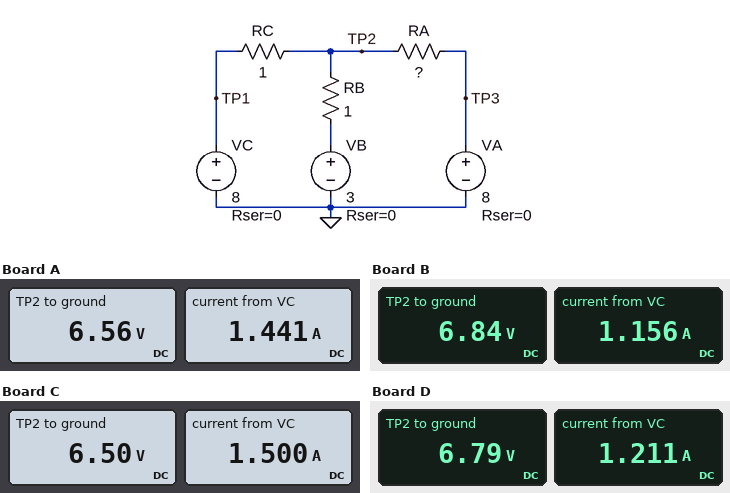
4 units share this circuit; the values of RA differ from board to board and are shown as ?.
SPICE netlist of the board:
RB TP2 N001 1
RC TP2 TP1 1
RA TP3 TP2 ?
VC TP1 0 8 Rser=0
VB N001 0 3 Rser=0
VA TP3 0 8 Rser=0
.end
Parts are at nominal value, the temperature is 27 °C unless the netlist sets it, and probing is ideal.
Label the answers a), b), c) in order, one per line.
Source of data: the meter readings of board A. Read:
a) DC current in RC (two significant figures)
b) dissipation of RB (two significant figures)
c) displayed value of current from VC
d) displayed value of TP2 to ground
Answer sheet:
a) 1.4 A
b) 13 W
c) 1.441 A
d) 6.56 V
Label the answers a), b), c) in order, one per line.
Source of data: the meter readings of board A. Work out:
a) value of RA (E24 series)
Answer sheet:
a) 0.68 Ω
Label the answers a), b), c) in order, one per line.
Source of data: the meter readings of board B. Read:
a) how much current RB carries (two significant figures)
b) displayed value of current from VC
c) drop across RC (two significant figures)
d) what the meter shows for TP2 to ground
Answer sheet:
a) 3.8 A
b) 1.156 A
c) 1.2 V
d) 6.84 V
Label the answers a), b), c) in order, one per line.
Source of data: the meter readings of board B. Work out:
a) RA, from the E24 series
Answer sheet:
a) 0.43 Ω
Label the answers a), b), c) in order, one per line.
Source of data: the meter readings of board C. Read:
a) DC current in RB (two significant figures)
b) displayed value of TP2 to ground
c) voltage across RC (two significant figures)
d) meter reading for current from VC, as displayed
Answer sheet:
a) 3.5 A
b) 6.50 V
c) 1.5 V
d) 1.500 A
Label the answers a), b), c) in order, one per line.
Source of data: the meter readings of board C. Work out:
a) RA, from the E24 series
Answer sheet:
a) 0.75 Ω
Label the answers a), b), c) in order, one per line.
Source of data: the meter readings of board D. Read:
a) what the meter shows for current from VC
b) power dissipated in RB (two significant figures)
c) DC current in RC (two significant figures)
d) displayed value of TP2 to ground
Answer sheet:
a) 1.211 A
b) 14 W
c) 1.2 A
d) 6.79 V
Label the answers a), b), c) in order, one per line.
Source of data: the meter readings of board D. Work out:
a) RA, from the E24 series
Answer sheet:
a) 0.47 Ω
